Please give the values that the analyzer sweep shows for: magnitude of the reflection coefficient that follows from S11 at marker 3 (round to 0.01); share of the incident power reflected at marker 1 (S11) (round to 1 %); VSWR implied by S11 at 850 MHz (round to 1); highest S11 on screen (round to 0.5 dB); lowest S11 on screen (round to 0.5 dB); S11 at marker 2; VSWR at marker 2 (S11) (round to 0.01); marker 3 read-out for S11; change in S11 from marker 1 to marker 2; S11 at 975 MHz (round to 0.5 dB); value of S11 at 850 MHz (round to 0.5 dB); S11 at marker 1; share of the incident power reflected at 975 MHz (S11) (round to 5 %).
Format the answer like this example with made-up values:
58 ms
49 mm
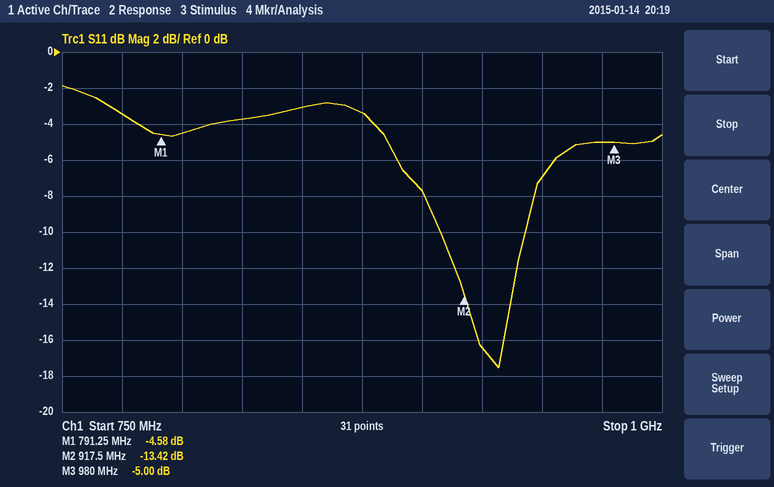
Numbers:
0.56
35 %
6
-2.0 dB
-17.5 dB
-13.42 dB
1.54
-5.00 dB
-8.84 dB
-5.0 dB
-3.0 dB
-4.58 dB
30 %
